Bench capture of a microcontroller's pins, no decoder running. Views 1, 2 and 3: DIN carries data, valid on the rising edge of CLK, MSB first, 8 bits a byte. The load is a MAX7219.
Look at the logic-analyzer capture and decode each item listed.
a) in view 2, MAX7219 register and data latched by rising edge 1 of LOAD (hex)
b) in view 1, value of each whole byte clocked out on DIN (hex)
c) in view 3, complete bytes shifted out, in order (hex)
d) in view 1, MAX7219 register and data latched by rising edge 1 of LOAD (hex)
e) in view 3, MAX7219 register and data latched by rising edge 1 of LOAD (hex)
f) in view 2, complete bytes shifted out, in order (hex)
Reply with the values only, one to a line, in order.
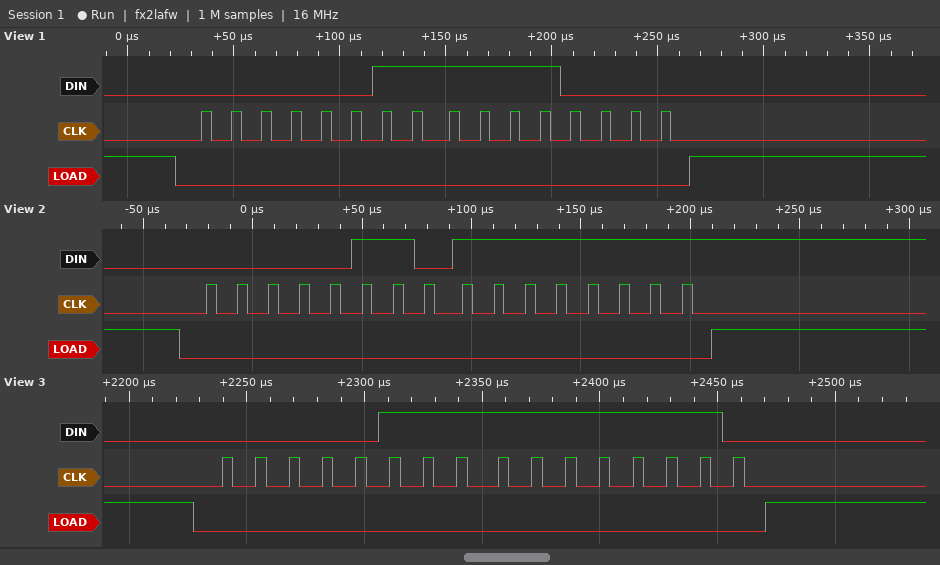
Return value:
register 0x6, data 0xFF
0x03 0xF0
07 FE
register 0x3, data 0xF0
register 0x7, data 0xFE
06 FF
